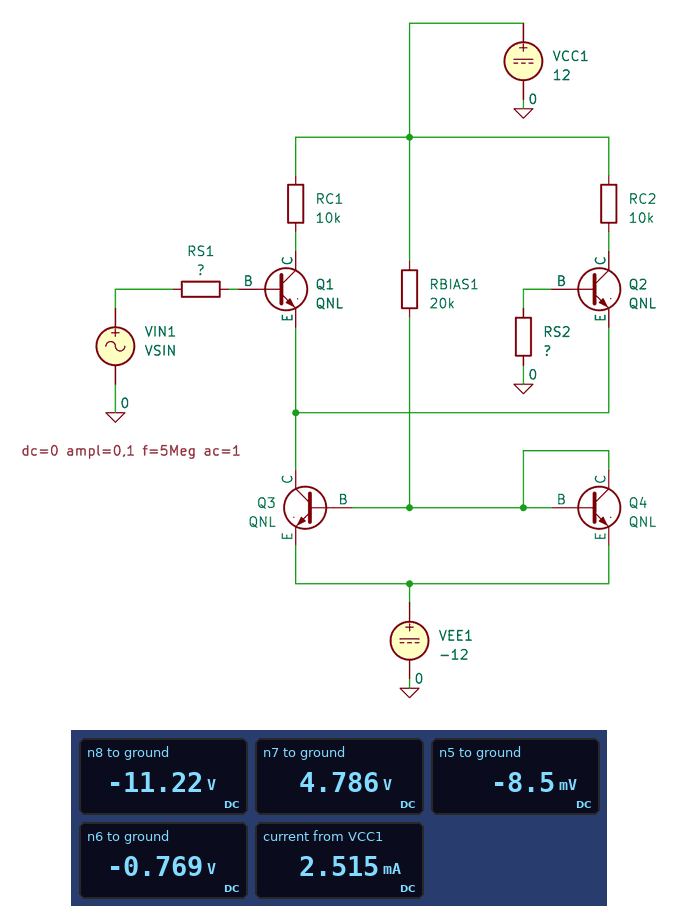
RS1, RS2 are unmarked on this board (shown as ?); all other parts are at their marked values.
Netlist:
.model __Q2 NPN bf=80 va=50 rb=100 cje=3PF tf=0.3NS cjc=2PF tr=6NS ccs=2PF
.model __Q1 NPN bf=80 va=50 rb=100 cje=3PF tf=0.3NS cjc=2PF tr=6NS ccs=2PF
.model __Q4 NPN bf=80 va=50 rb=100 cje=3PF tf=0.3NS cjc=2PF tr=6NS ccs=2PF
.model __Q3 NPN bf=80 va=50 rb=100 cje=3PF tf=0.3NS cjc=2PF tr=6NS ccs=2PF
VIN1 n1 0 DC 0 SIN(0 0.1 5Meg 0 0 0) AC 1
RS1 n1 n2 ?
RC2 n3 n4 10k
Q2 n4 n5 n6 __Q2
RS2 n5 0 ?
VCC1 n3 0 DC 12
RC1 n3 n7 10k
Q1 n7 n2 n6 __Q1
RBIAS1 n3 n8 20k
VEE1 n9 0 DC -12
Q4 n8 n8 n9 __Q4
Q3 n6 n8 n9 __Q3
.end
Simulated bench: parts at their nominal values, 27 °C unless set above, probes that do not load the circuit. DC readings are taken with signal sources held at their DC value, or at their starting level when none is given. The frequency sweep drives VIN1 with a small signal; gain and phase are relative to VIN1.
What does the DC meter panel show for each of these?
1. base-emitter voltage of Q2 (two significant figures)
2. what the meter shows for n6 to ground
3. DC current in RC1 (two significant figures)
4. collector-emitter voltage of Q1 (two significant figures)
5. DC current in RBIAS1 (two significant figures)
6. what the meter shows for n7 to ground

760 mV
-0.769 V
720 µA
5.6 V
1.2 mA
4.786 V
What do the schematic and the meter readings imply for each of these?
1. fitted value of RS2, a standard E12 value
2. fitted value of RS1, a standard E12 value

1.2 kΩ
560 Ω
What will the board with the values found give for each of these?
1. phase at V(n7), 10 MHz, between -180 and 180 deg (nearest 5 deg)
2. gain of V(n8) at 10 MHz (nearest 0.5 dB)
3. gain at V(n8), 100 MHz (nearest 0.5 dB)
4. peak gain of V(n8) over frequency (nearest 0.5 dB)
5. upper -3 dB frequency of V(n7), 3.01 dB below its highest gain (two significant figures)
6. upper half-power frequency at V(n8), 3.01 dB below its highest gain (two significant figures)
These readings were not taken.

95 deg
-62.5 dB
-48.0 dB
-47.5 dB
750 kHz
310 MHz
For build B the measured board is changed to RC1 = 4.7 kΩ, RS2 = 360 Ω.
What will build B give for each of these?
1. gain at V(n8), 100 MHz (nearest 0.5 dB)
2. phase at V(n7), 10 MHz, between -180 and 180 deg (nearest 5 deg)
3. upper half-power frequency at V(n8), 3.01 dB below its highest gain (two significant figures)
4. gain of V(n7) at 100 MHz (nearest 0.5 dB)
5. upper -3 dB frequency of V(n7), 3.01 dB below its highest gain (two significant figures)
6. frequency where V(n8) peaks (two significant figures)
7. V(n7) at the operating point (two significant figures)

-50.0 dB
110 deg
360 MHz
1.0 dB
1.6 MHz
170 MHz
8.8 V
